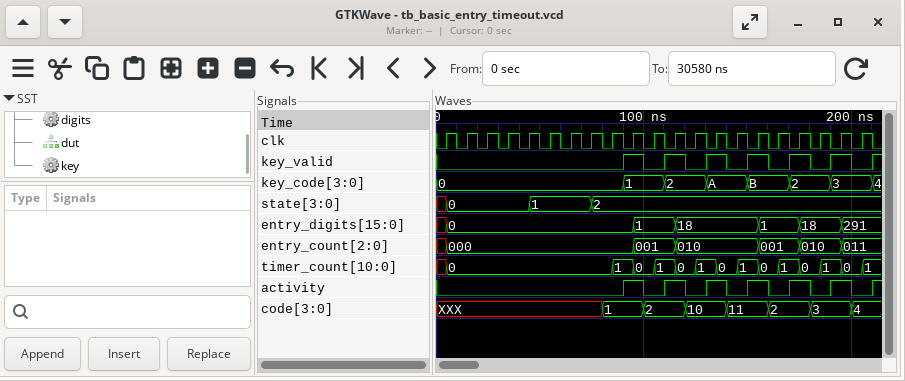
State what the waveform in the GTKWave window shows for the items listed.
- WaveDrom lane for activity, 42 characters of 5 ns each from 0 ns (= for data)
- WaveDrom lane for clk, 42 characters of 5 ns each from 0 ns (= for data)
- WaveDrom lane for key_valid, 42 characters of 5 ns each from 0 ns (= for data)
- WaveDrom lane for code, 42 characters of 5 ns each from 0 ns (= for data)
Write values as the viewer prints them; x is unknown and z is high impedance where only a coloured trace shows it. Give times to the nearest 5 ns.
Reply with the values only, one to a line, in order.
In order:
{name: 'activity', wave: '0.................1.0.1.0.1.0.1.0.1.0.1.0.'}
{name: 'clk', wave: '010101010101010101010101010101010101010101'}
{name: 'key_valid', wave: '0.................1.0.1.0.1.0.1.0.1.0.1.0.'}
{name: 'code', wave: 'x...............=...=...=...=...=...=...=.', data: '1 2 10 11 2 3 4'}
